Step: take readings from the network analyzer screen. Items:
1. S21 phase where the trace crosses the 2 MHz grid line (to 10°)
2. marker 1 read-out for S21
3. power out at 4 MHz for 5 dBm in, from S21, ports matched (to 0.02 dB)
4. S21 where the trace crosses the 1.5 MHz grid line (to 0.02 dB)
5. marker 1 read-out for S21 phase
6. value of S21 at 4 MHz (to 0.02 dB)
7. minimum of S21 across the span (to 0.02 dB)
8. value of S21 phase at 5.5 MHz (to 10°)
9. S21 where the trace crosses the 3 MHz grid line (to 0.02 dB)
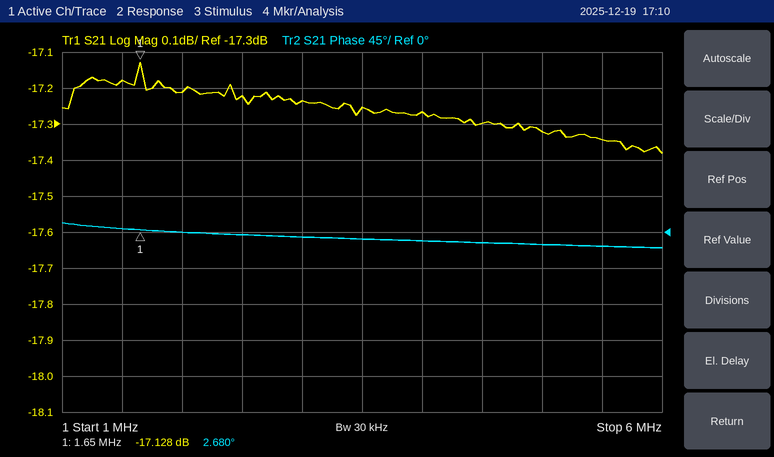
0°
-17.128 dB
-12.26 dBm
-17.18 dB
2.680°
-17.26 dB
-17.38 dB
-20°
-17.24 dB
